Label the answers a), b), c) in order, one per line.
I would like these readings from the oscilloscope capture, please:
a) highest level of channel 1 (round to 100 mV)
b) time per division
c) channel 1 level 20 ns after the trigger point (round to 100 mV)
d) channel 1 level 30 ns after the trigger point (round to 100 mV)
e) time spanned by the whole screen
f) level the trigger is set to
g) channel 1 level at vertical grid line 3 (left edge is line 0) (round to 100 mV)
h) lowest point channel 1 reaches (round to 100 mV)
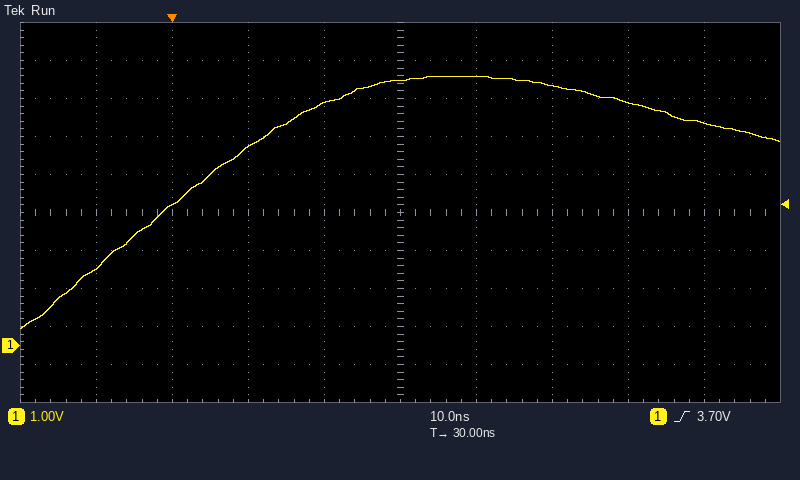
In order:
a) 7.1 V
b) 10 ns
c) 6.4 V
d) 7.0 V
e) 100 ns
f) 3.70 V
g) 5.2 V
h) 400 mV
